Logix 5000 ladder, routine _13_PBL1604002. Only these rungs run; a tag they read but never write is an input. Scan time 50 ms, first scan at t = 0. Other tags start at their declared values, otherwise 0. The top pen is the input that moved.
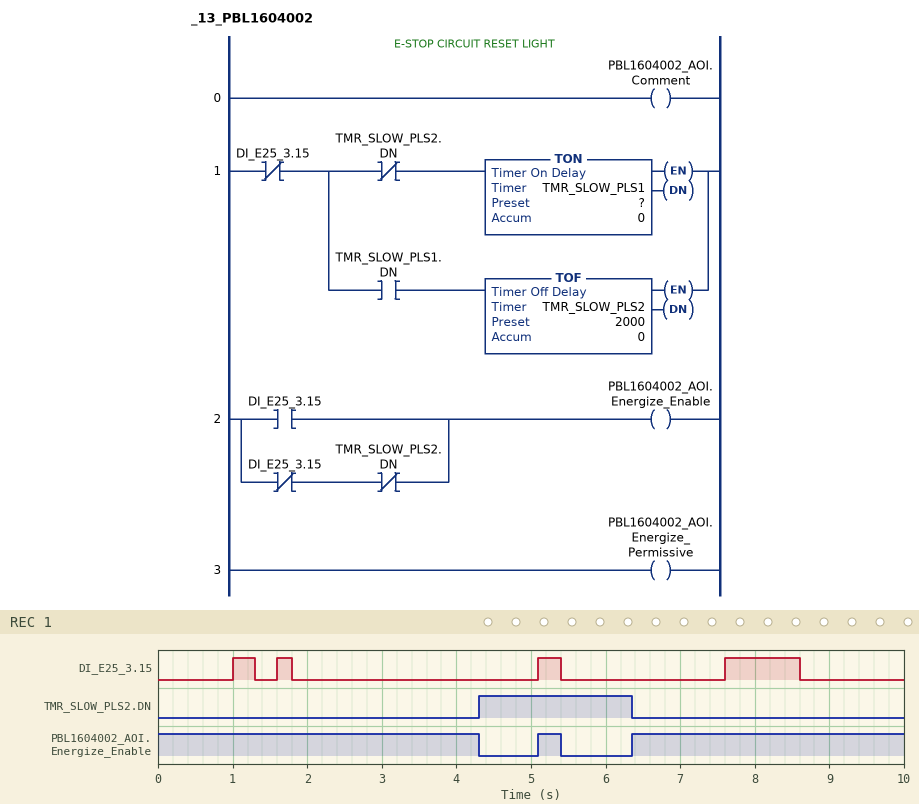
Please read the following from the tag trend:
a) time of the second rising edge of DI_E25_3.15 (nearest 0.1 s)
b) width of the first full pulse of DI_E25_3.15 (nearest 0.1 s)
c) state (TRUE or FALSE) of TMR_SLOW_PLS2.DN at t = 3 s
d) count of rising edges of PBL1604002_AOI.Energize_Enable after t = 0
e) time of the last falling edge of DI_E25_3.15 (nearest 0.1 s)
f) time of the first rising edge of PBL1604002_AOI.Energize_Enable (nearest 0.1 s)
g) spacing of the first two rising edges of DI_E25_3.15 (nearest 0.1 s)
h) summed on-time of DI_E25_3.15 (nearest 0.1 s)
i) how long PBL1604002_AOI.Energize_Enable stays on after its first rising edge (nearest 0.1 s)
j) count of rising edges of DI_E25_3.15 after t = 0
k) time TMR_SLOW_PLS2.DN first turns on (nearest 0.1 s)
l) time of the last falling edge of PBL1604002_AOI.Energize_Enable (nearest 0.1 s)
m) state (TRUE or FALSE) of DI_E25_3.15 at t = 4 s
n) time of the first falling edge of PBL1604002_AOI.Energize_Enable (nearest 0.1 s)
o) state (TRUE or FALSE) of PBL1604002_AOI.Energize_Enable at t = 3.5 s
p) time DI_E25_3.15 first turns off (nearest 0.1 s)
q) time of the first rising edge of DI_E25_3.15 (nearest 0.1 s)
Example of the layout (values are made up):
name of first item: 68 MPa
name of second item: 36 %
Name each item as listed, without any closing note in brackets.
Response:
time of the second rising edge of DI_E25_3.15: 1.6 s
width of the first full pulse of DI_E25_3.15: 0.3 s
state (TRUE or FALSE) of TMR_SLOW_PLS2.DN at t = 3 s: FALSE
count of rising edges of PBL1604002_AOI.Energize_Enable after t = 0: 2
time of the last falling edge of DI_E25_3.15: 8.6 s
time of the first rising edge of PBL1604002_AOI.Energize_Enable: 5.1 s
spacing of the first two rising edges of DI_E25_3.15: 0.6 s
summed on-time of DI_E25_3.15: 1.8 s
how long PBL1604002_AOI.Energize_Enable stays on after its first rising edge: 0.3 s
count of rising edges of DI_E25_3.15 after t = 0: 4
time TMR_SLOW_PLS2.DN first turns on: 4.3 s
time of the last falling edge of PBL1604002_AOI.Energize_Enable: 5.4 s
state (TRUE or FALSE) of DI_E25_3.15 at t = 4 s: FALSE
time of the first falling edge of PBL1604002_AOI.Energize_Enable: 4.3 s
state (TRUE or FALSE) of PBL1604002_AOI.Energize_Enable at t = 3.5 s: TRUE
time DI_E25_3.15 first turns off: 1.3 s
time of the first rising edge of DI_E25_3.15: 1.0 s
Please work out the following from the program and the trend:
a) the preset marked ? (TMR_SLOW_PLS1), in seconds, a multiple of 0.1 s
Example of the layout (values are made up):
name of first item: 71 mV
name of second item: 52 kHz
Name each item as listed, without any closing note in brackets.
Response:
the preset marked ? (TMR_SLOW_PLS1), in seconds, a multiple of 0.1 s: 2.5 s
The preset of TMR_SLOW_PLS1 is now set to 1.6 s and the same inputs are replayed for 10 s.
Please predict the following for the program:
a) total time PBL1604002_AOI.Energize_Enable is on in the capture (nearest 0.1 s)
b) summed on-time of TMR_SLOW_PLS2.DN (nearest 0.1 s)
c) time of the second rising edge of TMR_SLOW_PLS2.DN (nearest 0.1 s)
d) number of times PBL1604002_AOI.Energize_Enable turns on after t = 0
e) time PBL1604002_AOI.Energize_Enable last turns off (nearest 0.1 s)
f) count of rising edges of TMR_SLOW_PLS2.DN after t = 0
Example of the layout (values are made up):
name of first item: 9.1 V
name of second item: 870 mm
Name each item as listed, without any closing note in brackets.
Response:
total time PBL1604002_AOI.Energize_Enable is on in the capture: 7.2 s
summed on-time of TMR_SLOW_PLS2.DN: 4.1 s
time of the second rising edge of TMR_SLOW_PLS2.DN: 7.1 s
number of times PBL1604002_AOI.Energize_Enable turns on after t = 0: 4
time PBL1604002_AOI.Energize_Enable last turns off: 8.6 s
count of rising edges of TMR_SLOW_PLS2.DN after t = 0: 2
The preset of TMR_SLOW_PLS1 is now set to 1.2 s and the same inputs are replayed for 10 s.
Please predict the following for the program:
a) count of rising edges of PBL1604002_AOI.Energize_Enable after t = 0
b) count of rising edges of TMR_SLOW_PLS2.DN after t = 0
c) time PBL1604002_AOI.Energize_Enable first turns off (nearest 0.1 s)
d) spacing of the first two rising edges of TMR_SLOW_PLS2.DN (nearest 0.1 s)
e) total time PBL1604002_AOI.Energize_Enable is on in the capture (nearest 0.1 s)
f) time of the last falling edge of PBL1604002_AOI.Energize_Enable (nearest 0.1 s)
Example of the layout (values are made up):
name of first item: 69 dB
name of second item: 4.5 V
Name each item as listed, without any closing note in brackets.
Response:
count of rising edges of PBL1604002_AOI.Energize_Enable after t = 0: 3
count of rising edges of TMR_SLOW_PLS2.DN after t = 0: 3
time PBL1604002_AOI.Energize_Enable first turns off: 3.0 s
spacing of the first two rising edges of TMR_SLOW_PLS2.DN: 3.6 s
total time PBL1604002_AOI.Energize_Enable is on in the capture: 6.8 s
time of the last falling edge of PBL1604002_AOI.Energize_Enable: 9.9 s
